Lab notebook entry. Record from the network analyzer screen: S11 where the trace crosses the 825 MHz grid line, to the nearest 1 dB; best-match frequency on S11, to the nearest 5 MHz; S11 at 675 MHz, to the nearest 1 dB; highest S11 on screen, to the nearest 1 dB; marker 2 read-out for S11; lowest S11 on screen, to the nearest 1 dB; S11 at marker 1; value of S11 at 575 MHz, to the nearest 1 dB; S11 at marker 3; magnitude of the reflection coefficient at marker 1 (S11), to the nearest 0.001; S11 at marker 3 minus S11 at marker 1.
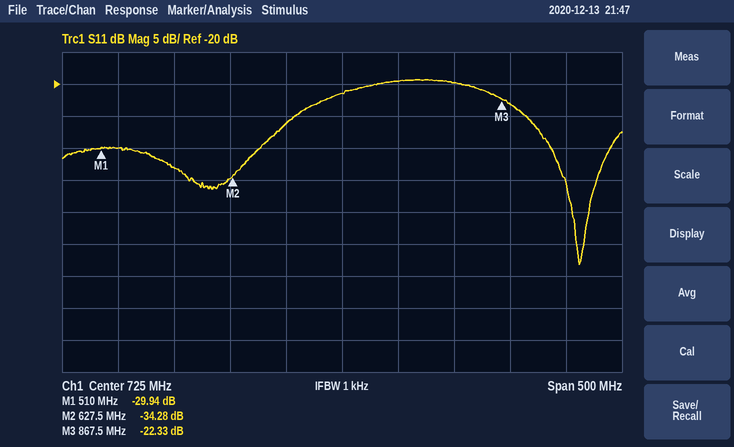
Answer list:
-20 dB
935 MHz
-26 dB
-19 dB
-34.28 dB
-48 dB
-29.94 dB
-33 dB
-22.33 dB
0.032
7.61 dB
